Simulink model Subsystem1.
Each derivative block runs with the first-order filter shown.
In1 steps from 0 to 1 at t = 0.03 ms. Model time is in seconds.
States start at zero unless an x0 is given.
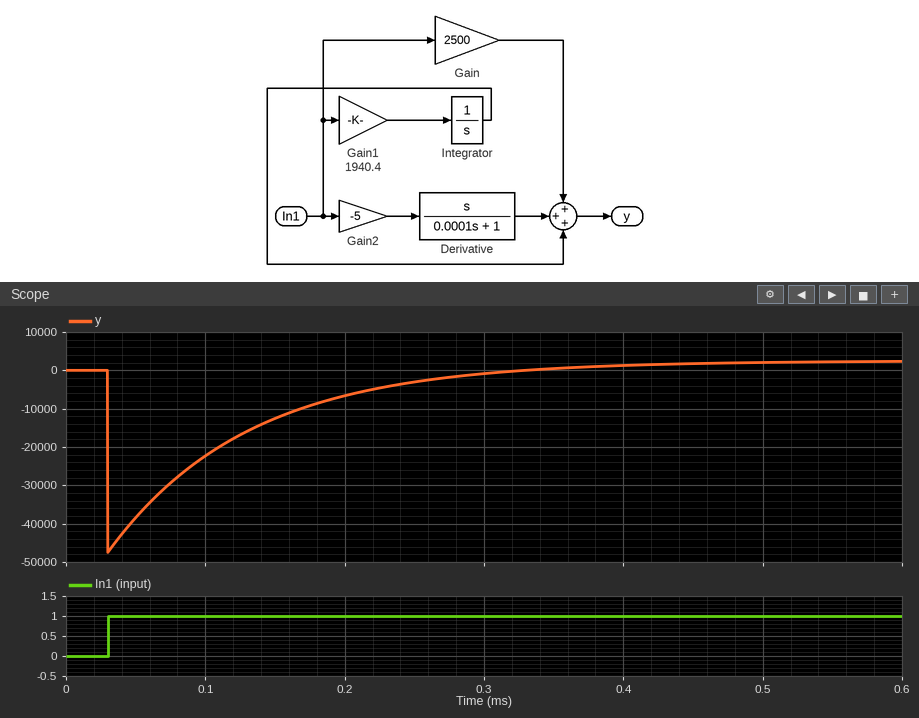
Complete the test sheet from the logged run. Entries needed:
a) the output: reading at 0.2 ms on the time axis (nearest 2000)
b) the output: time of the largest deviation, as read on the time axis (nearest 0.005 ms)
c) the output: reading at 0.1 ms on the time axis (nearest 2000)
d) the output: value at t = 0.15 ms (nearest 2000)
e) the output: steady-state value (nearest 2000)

-6000
0.030 ms
-22000
-12000
2000
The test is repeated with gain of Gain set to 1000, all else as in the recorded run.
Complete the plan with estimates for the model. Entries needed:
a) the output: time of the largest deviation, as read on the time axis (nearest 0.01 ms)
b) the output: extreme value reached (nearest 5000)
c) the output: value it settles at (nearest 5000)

0.03 ms
-50000
0
